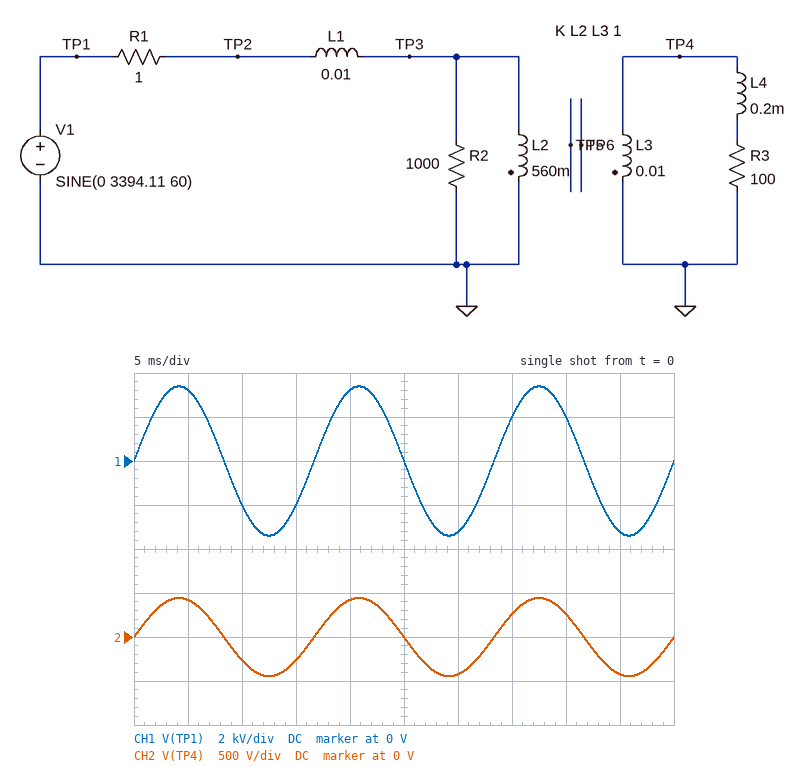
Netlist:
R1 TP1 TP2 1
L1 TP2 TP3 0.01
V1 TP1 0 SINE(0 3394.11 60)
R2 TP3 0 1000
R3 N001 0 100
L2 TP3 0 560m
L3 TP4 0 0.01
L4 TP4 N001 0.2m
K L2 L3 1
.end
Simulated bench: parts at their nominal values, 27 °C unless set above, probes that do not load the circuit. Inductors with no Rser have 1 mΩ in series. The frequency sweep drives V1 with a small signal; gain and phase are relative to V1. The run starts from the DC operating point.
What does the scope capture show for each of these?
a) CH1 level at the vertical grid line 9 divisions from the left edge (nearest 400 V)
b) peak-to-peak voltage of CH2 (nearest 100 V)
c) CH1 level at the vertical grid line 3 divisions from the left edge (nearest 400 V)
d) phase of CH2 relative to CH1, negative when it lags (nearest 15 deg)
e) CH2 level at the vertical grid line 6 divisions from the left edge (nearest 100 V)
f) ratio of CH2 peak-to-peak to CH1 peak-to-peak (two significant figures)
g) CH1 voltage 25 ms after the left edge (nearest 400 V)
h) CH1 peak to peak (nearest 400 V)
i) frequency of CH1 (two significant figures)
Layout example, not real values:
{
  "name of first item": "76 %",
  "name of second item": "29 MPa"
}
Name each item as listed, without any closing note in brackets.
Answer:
{
  "CH1 level at the vertical grid line 9 divisions from the left edge": "-3.2 kV",
  "peak-to-peak voltage of CH2": "900 V",
  "CH1 level at the vertical grid line 3 divisions from the left edge": "-2.0 kV",
  "phase of CH2 relative to CH1, negative when it lags": "0 deg",
  "CH2 level at the vertical grid line 6 divisions from the left edge": "-400 V",
  "ratio of CH2 peak-to-peak to CH1 peak-to-peak": "0.13",
  "CH1 voltage 25 ms after the left edge": "0 V",
  "CH1 peak to peak": "6.8 kV",
  "frequency of CH1": "60 Hz"
}
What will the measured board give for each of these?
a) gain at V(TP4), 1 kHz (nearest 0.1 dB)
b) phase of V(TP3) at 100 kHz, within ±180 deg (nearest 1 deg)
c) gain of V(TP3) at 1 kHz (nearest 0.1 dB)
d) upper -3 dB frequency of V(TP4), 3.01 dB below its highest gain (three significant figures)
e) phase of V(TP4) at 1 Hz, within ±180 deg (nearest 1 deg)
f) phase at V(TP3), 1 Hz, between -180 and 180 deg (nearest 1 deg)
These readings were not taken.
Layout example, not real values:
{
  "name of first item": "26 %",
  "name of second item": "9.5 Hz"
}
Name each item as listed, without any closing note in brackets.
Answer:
{
  "gain at V(TP4), 1 kHz": "-17.7 dB",
  "phase of V(TP3) at 100 kHz, within ±180 deg": "-77 deg",
  "gain of V(TP3) at 1 kHz": "-0.2 dB",
  "upper -3 dB frequency of V(TP4), 3.01 dB below its highest gain": "13.5 kHz",
  "phase of V(TP4) at 1 Hz, within ±180 deg": "16 deg",
  "phase at V(TP3), 1 Hz, between -180 and 180 deg": "16 deg"
}
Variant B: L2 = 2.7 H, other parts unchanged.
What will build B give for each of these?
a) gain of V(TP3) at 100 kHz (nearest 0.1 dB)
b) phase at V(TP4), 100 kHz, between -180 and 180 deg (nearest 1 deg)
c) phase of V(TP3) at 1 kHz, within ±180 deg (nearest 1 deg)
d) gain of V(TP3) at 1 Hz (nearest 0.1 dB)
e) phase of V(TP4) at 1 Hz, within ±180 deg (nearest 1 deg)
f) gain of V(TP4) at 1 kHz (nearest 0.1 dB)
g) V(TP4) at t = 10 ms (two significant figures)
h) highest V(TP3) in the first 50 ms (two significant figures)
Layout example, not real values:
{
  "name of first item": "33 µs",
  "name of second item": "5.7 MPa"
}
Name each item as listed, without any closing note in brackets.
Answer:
{
  "gain of V(TP3) at 100 kHz": "-16.2 dB",
  "phase at V(TP4), 100 kHz, between -180 and 180 deg": "-80 deg",
  "phase of V(TP3) at 1 kHz, within ±180 deg": "-4 deg",
  "gain of V(TP3) at 1 Hz": "-0.1 dB",
  "phase of V(TP4) at 1 Hz, within ±180 deg": "3 deg",
  "gain of V(TP4) at 1 kHz": "-24.4 dB",
  "V(TP4) at t = 10 ms": "-120 V",
  "highest V(TP3) in the first 50 ms": "3.4 kV"
}
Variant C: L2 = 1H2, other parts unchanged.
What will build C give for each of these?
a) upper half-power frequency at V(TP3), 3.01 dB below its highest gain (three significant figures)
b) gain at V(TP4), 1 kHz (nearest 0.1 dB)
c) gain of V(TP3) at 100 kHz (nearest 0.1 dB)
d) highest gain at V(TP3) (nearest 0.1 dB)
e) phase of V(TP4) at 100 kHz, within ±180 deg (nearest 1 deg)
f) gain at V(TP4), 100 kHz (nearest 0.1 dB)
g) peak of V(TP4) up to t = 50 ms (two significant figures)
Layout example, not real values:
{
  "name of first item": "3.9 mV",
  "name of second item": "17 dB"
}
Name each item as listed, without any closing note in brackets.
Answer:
{
  "upper half-power frequency at V(TP3), 3.01 dB below its highest gain": "14.7 kHz",
  "gain at V(TP4), 1 kHz": "-20.9 dB",
  "gain of V(TP3) at 100 kHz": "-16.4 dB",
  "highest gain at V(TP3)": "-0.1 dB",
  "phase of V(TP4) at 100 kHz, within ±180 deg": "-79 deg",
  "gain at V(TP4), 100 kHz": "-37.2 dB",
  "peak of V(TP4) up to t = 50 ms": "310 V"
}
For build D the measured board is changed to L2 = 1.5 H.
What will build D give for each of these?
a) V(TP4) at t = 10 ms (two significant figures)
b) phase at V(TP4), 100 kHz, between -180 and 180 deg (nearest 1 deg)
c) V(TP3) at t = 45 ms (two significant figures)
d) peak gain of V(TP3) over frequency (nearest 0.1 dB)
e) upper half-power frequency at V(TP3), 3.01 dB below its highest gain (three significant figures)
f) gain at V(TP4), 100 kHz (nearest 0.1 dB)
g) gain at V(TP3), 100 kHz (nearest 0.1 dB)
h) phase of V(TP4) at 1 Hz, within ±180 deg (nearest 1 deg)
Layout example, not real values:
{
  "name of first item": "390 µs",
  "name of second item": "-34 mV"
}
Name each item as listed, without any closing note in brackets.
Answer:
{
  "V(TP4) at t = 10 ms": "-160 V",
  "phase at V(TP4), 100 kHz, between -180 and 180 deg": "-79 deg",
  "V(TP3) at t = 45 ms": "-3.2 kV",
  "peak gain of V(TP3) over frequency": "-0.1 dB",
  "upper half-power frequency at V(TP3), 3.01 dB below its highest gain": "14.9 kHz",
  "gain at V(TP4), 100 kHz": "-38.1 dB",
  "gain at V(TP3), 100 kHz": "-16.3 dB",
  "phase of V(TP4) at 1 Hz, within ±180 deg": "6 deg"
}
